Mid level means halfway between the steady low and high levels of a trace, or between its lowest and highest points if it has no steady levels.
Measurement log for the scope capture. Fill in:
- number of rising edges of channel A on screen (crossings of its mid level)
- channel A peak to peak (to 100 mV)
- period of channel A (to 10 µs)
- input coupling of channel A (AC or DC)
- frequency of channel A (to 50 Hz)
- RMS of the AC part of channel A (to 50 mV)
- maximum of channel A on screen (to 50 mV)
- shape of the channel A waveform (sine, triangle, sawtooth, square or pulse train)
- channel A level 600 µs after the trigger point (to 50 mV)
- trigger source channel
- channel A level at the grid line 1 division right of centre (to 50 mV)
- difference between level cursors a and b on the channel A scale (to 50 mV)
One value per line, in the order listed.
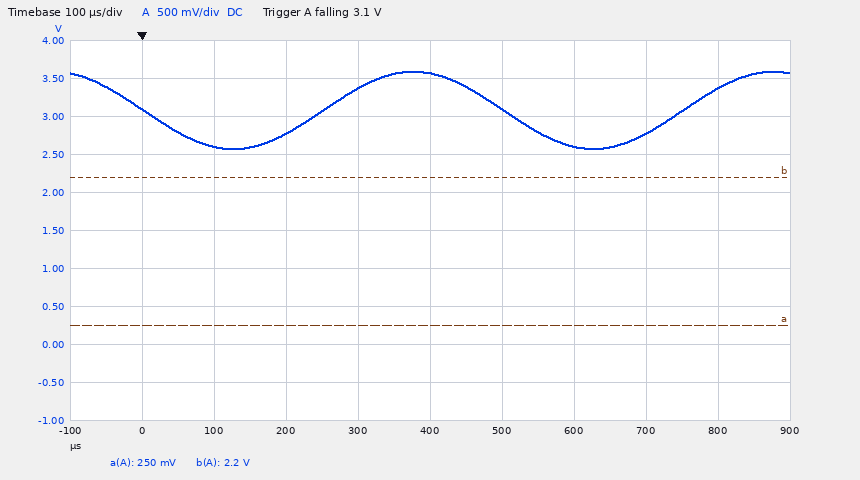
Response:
2
1.00 V
500 µs
DC
2.00 kHz
350 mV
3.60 V
sine
2.60 V
channel A
3.10 V
1.95 V
